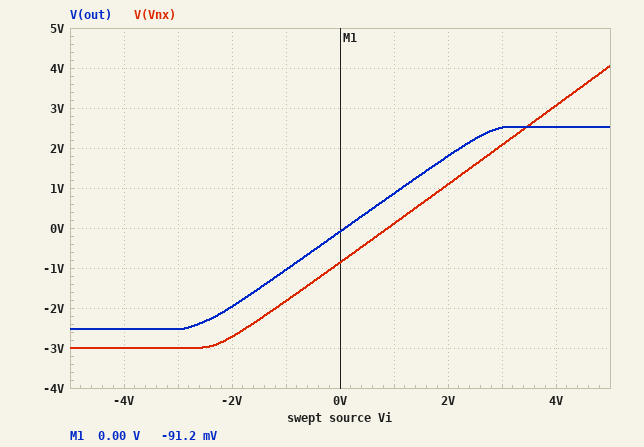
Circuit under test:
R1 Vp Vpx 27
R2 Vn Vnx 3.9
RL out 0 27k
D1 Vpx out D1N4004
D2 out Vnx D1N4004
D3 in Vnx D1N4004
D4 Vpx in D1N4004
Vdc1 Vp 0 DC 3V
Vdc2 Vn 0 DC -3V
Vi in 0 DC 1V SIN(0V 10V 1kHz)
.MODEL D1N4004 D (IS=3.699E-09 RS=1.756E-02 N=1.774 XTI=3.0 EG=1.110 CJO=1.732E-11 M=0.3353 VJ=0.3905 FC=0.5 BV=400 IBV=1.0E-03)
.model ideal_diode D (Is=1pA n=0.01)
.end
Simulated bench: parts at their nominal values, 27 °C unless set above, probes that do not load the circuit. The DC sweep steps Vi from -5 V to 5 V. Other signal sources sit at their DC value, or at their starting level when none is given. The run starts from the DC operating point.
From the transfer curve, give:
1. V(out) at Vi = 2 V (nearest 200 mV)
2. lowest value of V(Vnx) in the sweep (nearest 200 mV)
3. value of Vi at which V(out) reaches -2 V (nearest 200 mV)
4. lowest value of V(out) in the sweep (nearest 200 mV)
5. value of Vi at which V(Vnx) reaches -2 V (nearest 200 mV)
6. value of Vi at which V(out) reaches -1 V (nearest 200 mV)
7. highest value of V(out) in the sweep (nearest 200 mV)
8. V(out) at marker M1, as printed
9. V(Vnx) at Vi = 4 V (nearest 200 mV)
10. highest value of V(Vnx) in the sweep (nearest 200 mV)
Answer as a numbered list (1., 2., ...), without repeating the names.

1. 1.8 V
2. -3.0 V
3. -2.0 V
4. -2.6 V
5. -1.2 V
6. -1.0 V
7. 2.6 V
8. -91.2 mV
9. 3.0 V
10. 4.0 V
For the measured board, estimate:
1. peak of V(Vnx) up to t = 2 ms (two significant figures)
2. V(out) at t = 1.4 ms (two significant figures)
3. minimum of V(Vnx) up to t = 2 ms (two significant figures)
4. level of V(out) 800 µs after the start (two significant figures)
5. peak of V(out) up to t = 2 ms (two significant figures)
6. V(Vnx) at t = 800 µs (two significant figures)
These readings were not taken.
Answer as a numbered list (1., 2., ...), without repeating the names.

1. 9.0 V
2. 2.5 V
3. -3.0 V
4. -2.5 V
5. 2.5 V
6. -3.0 V
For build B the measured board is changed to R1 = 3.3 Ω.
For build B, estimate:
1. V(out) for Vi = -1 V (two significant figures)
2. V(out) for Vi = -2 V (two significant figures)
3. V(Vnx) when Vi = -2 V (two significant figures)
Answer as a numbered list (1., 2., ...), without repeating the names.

1. -940 mV
2. -1.9 V
3. -2.6 V
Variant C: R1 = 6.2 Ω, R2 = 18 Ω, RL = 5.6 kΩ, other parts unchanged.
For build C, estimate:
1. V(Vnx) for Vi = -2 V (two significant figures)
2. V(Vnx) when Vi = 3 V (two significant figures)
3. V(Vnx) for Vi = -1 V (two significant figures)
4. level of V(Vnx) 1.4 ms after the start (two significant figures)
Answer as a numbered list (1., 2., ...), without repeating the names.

1. -2.6 V
2. 2.2 V
3. -1.7 V
4. 5.0 V
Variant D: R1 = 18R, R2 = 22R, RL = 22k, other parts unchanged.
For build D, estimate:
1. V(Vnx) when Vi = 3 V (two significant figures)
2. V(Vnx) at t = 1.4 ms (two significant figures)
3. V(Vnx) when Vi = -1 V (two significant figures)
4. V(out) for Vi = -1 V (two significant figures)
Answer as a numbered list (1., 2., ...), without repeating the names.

1. 2.2 V
2. 5.0 V
3. -1.7 V
4. -950 mV
